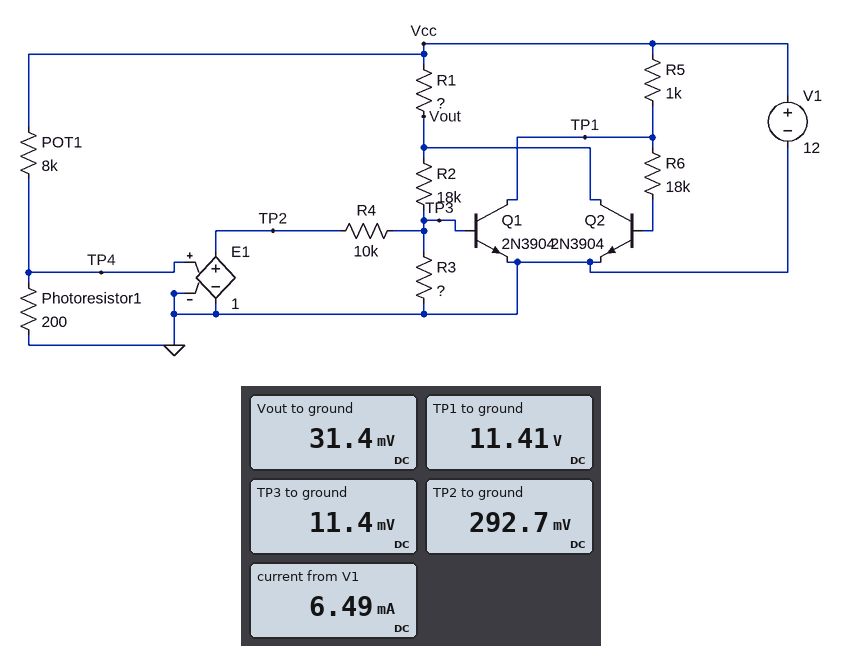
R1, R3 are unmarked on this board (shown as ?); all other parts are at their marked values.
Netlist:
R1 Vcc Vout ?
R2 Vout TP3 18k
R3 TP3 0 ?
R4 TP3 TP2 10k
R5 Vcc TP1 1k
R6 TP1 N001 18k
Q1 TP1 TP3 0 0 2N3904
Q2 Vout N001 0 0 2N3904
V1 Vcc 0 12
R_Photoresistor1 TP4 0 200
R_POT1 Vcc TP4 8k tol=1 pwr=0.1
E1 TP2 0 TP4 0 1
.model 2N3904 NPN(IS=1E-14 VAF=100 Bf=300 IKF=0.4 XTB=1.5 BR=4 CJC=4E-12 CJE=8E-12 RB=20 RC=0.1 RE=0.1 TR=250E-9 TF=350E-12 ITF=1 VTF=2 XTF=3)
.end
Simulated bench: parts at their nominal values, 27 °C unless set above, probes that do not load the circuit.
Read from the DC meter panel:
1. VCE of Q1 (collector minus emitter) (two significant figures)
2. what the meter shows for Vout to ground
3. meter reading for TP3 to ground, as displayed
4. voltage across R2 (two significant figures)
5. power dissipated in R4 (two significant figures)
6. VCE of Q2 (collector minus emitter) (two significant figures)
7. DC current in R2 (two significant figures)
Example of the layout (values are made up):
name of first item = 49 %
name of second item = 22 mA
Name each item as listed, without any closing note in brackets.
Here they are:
VCE of Q1 (collector minus emitter) = 11 V
what the meter shows for Vout to ground = 31.4 mV
meter reading for TP3 to ground, as displayed = 11.4 mV
voltage across R2 = 20 mV
power dissipated in R4 = 7.9 µW
VCE of Q2 (collector minus emitter) = 31 mV
DC current in R2 = 1.1 µA
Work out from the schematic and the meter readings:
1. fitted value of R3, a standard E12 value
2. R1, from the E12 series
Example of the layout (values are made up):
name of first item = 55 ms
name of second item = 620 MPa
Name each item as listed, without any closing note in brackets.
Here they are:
fitted value of R3, a standard E12 value = 390 Ω
R1, from the E12 series = 2.7 kΩ
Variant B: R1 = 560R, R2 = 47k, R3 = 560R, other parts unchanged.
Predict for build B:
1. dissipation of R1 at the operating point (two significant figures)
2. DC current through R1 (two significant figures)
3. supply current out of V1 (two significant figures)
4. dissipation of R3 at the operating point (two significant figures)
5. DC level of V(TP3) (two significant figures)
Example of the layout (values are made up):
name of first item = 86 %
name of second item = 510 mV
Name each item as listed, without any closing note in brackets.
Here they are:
dissipation of R1 at the operating point = 250 mW
DC current through R1 = 21 mA
supply current out of V1 = 23 mA
dissipation of R3 at the operating point = 460 nW
DC level of V(TP3) = 16 mV
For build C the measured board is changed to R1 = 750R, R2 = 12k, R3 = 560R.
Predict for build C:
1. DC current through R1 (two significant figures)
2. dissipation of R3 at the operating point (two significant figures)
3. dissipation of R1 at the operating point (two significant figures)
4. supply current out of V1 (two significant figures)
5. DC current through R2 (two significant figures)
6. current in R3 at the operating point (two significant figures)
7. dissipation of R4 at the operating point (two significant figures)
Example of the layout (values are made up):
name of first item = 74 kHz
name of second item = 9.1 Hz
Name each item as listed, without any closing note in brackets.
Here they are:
DC current through R1 = 16 mA
dissipation of R3 at the operating point = 540 nW
dissipation of R1 at the operating point = 190 mW
supply current out of V1 = 18 mA
DC current through R2 = 3.6 µA
current in R3 at the operating point = 31 µA
dissipation of R4 at the operating point = 7.6 µW
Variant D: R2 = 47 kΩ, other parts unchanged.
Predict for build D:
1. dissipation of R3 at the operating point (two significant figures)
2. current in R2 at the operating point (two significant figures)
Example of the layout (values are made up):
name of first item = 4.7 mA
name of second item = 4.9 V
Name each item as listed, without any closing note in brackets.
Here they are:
dissipation of R3 at the operating point = 320 nW
current in R2 at the operating point = 430 nA
